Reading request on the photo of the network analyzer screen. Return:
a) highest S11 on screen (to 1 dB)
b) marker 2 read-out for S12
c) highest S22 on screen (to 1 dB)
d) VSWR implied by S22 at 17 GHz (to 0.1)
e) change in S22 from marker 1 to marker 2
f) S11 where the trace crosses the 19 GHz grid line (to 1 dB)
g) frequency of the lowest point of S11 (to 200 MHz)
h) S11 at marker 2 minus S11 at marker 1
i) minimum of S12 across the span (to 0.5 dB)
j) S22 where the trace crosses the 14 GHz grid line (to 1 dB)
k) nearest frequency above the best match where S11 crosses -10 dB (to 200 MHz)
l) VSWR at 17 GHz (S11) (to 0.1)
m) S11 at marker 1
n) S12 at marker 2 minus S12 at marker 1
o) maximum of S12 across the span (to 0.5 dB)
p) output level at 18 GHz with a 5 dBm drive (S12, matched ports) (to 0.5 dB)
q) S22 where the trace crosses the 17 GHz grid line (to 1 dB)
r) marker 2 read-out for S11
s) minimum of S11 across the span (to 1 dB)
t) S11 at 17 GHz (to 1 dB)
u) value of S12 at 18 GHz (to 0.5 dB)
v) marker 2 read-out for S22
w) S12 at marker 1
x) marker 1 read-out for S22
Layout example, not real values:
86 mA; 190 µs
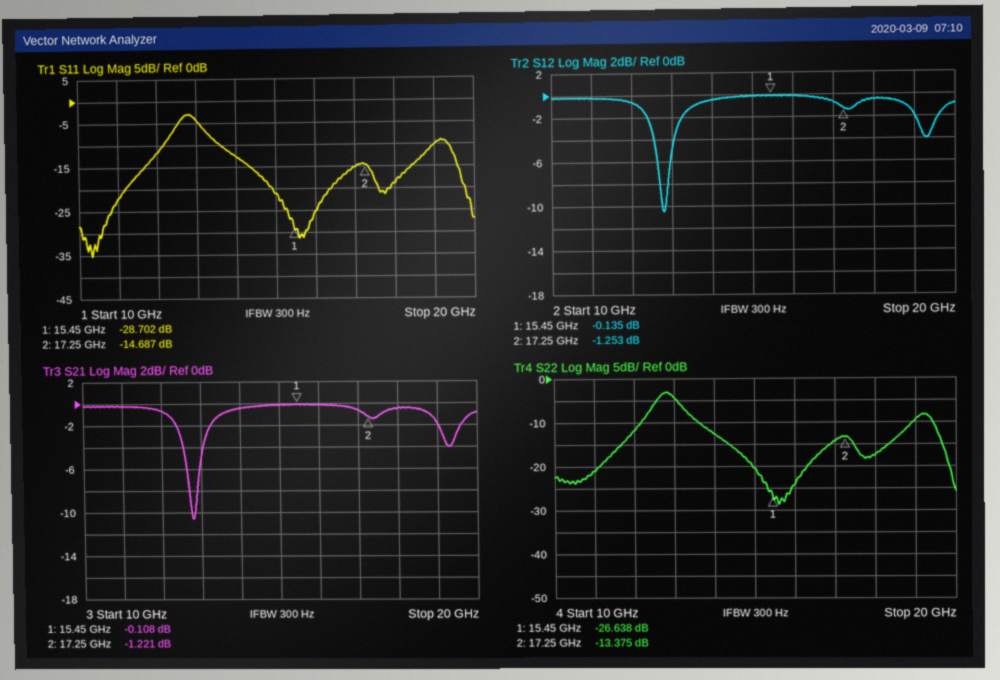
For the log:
-3 dB; -1.253 dB; -3 dB; 1.5; 13.263 dB; -10 dB; 10.4 GHz; 14.015 dB; -10.5 dB; -13 dB; 12.2 GHz; 1.4; -28.702 dB; -1.118 dB; 0.0 dB; 4.5 dBm; -14 dB; -14.687 dB; -35 dB; -15 dB; -0.5 dB; -13.375 dB; -0.135 dB; -26.638 dB
